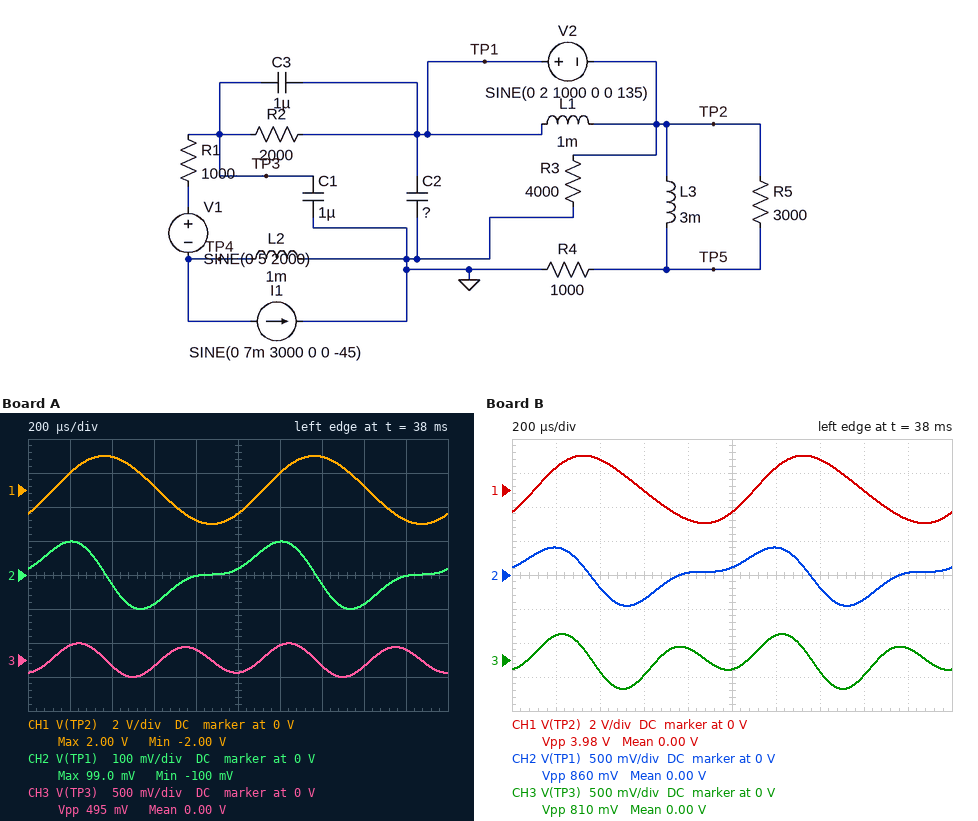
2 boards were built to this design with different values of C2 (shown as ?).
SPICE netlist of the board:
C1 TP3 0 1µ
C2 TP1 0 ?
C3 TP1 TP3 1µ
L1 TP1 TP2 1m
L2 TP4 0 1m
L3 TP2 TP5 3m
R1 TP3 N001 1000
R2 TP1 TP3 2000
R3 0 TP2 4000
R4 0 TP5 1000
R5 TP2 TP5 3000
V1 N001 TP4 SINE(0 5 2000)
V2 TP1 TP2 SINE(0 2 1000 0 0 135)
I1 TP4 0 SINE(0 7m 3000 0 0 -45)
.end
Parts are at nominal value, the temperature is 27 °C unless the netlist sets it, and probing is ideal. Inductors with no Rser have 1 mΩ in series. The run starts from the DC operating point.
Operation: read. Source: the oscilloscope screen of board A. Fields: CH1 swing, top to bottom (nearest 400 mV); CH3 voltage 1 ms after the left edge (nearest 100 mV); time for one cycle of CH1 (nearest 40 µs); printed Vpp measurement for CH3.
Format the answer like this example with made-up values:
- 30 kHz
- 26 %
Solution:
- 4.0 V
- -200 mV
- 1.00 ms
- 495 mV
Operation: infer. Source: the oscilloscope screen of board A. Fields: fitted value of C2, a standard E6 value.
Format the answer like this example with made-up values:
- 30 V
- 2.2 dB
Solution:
- 4.7 µF
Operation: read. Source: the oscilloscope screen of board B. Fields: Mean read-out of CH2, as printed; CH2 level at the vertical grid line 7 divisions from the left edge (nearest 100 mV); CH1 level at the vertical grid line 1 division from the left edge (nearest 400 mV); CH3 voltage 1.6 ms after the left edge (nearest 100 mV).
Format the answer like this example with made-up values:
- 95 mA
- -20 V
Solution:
- 0.00 V
- -200 mV
- 1.2 V
- -200 mV
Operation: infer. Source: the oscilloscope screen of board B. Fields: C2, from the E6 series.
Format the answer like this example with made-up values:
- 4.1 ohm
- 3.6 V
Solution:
- 680 nF
